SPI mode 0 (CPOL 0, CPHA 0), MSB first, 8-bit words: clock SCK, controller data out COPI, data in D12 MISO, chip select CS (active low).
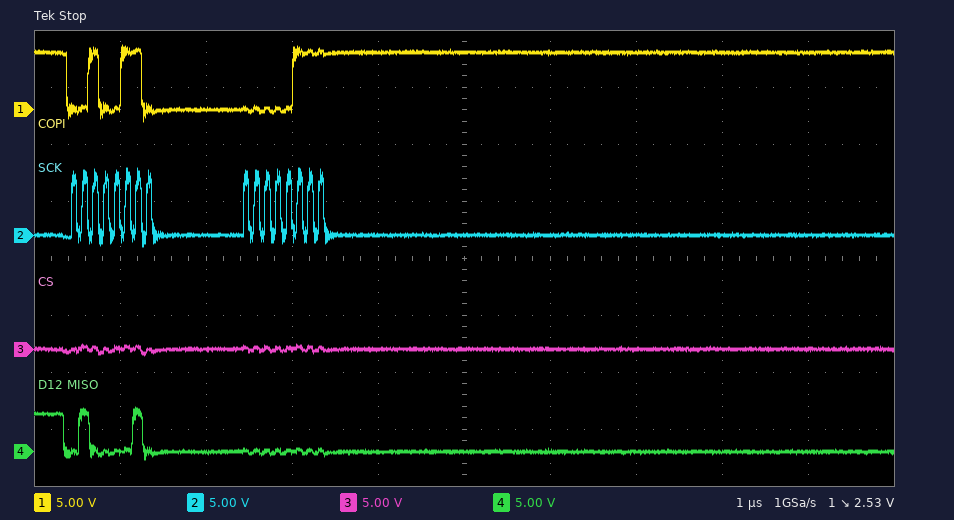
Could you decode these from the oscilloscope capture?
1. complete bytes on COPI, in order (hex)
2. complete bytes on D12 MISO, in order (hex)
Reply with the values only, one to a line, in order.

26 07
42 00
